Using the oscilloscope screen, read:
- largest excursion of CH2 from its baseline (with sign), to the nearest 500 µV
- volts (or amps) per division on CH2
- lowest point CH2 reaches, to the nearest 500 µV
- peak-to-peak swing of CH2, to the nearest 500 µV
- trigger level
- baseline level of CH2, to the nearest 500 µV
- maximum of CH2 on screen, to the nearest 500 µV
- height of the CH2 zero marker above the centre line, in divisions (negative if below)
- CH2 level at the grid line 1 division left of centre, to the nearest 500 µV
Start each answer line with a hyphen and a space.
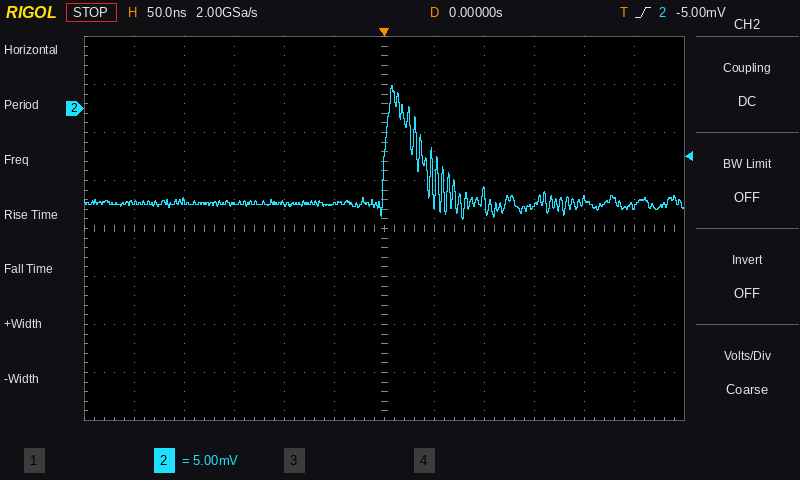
- +12.5 mV
- 5 mV
- -11.5 mV
- 14.0 mV
- -5.00 mV
- -10.0 mV
- 2.5 mV
- +2.5 div
- -10.0 mV
